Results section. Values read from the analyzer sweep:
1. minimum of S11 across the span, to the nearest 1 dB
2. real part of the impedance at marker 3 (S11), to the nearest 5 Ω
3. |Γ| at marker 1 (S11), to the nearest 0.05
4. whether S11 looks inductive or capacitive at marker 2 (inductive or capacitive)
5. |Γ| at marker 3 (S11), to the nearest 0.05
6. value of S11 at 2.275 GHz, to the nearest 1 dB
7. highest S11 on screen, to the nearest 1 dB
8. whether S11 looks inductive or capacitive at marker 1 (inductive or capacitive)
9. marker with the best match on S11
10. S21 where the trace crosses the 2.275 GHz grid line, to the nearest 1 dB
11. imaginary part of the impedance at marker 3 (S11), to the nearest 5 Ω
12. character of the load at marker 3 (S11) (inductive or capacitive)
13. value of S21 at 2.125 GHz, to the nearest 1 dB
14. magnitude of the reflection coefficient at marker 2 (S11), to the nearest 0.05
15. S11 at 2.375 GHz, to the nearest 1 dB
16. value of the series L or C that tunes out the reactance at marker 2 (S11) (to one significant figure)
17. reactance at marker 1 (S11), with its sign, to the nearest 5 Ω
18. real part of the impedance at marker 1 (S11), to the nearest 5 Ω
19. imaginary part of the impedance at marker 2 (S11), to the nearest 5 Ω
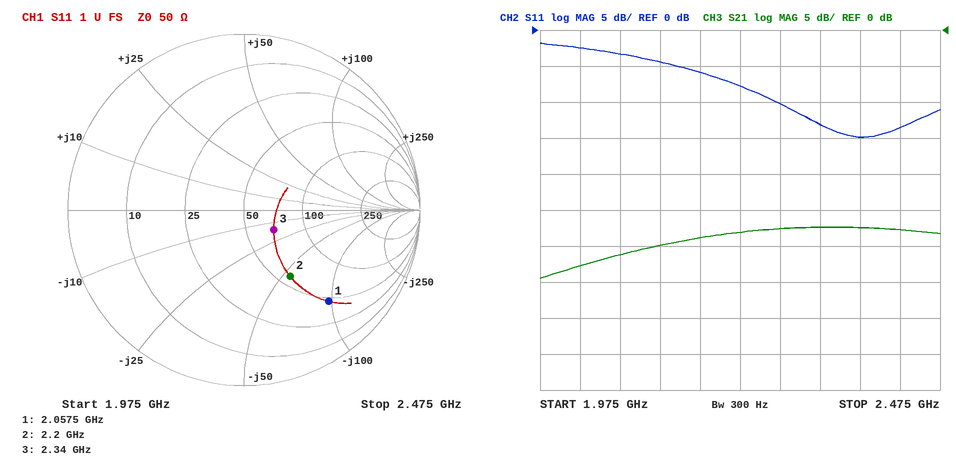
-15 dB
70 Ω
0.70
capacitive
0.20
-10 dB
-2 dB
capacitive
marker 3
-28 dB
-15 Ω
capacitive
-30 dB
0.45
-15 dB
4 nH
-95 Ω
45 Ω
-55 Ω
